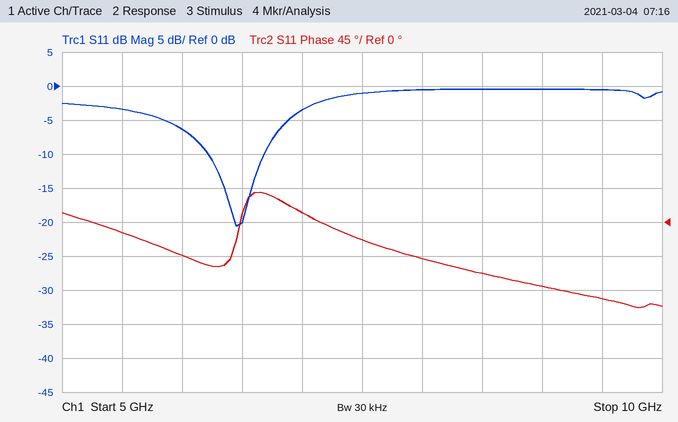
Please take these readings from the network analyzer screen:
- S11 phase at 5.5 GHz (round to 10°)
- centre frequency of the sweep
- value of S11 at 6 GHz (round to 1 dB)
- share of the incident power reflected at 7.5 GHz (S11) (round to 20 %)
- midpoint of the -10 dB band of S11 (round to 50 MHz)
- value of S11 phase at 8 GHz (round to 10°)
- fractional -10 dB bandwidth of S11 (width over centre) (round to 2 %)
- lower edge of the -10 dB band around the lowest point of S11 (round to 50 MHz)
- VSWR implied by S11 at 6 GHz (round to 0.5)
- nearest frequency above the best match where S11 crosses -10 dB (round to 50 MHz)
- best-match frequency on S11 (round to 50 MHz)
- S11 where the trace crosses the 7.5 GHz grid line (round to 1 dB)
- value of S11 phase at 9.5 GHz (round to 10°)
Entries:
-10°
7.5 GHz
-6 dB
80 %
6.45 GHz
-50°
8 %
6.20 GHz
3.0
6.70 GHz
6.45 GHz
-1 dB
-100°
